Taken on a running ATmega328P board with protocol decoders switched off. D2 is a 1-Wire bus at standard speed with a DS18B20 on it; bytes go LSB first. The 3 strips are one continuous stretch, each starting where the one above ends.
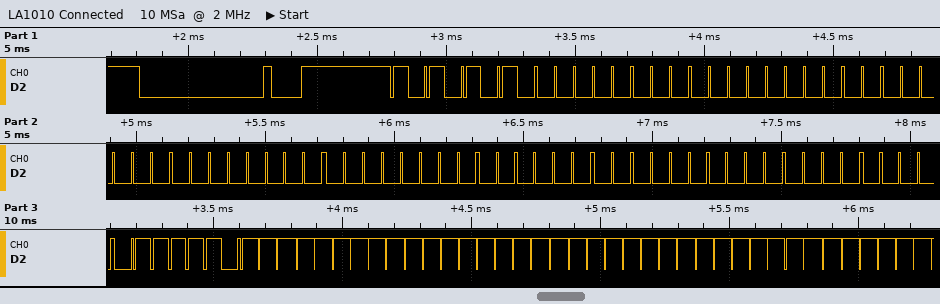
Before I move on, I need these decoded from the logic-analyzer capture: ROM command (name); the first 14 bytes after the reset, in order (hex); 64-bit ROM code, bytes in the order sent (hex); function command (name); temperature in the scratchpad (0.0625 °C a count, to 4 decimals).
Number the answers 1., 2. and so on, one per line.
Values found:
1. Match ROM
2. 55 00 00 00 00 00 00 00 00 BE FF FF FF FF
3. 00 00 00 00 00 00 00 00
4. Read Scratchpad
5. -0.0625 °C
